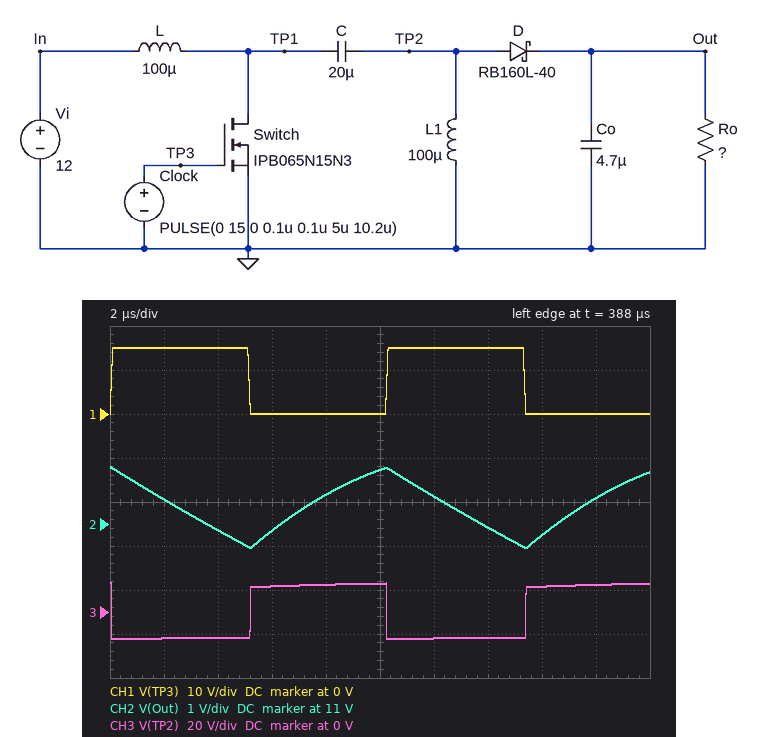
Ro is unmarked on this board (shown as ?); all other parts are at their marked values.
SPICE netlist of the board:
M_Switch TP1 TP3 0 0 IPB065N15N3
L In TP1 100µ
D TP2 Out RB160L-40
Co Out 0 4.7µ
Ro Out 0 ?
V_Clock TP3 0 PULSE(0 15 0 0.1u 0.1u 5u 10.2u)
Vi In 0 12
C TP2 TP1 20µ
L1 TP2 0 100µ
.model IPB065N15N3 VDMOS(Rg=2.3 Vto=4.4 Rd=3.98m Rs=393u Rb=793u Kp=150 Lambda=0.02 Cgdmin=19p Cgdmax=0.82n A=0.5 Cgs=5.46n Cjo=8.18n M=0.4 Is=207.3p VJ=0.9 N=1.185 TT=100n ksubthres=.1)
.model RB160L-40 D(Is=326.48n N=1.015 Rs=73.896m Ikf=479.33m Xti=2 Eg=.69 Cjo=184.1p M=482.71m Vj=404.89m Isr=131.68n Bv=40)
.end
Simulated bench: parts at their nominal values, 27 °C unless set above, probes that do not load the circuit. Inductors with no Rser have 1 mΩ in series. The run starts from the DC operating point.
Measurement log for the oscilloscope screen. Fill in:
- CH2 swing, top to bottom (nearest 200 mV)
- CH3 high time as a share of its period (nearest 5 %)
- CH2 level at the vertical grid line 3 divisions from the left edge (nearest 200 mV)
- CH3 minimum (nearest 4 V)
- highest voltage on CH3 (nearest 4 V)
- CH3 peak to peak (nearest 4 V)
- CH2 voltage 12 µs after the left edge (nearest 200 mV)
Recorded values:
1.8 V
50 %
10.8 V
-12 V
12 V
24 V
11.6 V
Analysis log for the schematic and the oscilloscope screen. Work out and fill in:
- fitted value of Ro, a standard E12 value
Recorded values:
6.8 Ω
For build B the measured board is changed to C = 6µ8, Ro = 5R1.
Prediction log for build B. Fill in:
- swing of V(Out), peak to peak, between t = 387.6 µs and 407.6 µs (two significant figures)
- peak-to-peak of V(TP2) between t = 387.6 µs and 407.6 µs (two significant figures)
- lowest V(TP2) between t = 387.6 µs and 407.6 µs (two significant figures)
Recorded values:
2.4 V
26 V
-13 V
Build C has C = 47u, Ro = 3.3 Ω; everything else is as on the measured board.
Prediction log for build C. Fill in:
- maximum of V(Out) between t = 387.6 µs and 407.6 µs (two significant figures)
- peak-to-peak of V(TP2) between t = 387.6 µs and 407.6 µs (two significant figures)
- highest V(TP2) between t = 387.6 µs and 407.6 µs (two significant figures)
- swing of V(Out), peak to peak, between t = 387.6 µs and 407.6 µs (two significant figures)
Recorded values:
13 V
26 V
14 V
3.6 V
